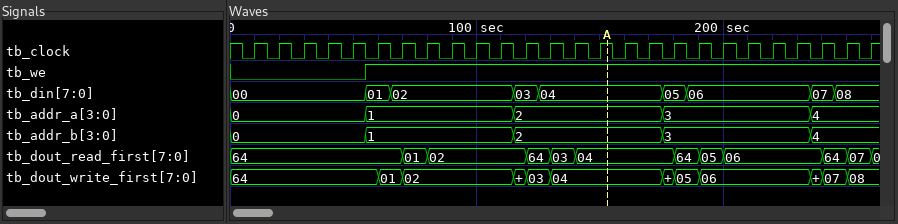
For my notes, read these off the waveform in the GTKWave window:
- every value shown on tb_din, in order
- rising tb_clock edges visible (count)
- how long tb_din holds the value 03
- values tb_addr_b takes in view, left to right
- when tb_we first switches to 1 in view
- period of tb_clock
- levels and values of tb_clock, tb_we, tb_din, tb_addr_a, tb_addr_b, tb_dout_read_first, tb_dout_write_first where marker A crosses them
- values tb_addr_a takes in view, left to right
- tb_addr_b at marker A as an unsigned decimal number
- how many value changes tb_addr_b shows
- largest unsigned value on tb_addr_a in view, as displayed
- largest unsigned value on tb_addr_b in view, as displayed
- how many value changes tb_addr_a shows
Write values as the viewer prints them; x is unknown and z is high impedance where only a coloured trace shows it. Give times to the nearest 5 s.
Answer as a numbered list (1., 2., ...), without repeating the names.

1. 00, 01, 02, 03, 04, 05, 06, 07, 08
2. 26
3. 10 s
4. 0, 1, 2, 3, 4
5. 55 s
6. 10 s
7. tb_clock=1, tb_we=1, tb_din=04, tb_addr_a=2, tb_addr_b=2, tb_dout_read_first=04, tb_dout_write_first=04
8. 0, 1, 2, 3, 4
9. 2
10. 4
11. 4
12. 4
13. 4
